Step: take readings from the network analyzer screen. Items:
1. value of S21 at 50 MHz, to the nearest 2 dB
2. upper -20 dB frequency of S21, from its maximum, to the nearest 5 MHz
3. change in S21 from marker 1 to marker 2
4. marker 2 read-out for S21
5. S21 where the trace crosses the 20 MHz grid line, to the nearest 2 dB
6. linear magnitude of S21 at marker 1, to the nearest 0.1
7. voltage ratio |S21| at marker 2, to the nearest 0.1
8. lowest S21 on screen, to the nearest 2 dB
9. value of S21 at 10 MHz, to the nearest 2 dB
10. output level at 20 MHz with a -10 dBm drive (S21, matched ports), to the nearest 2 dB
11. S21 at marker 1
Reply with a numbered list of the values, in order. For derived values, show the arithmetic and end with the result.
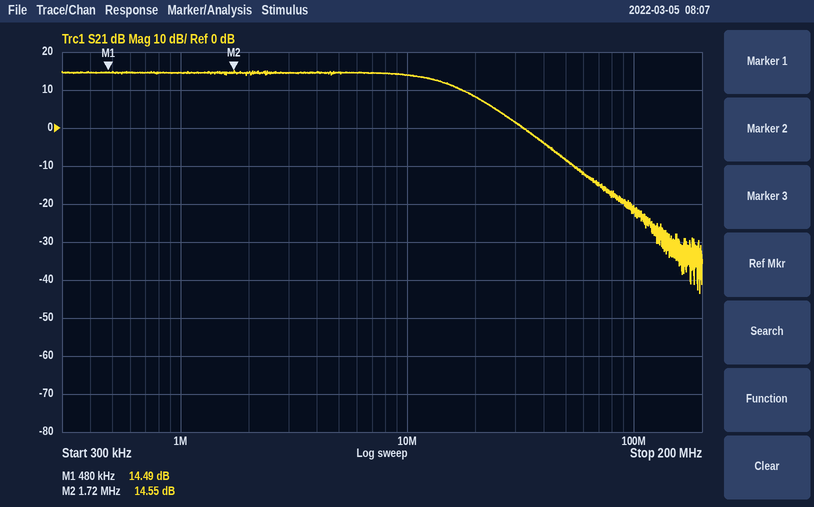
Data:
1. -8 dB
2. 40 MHz
3. 14.55 − (14.49) = 0.06 dB
4. 14.55 dB
5. 8 dB
6. 10^(14.49/20) ≈ 5.3
7. 10^(14.55/20) ≈ 5.3
8. -44 dB
9. 14 dB
10. -10 dBm + (8 dB) = -2 dBm
11. 14.49 dB
